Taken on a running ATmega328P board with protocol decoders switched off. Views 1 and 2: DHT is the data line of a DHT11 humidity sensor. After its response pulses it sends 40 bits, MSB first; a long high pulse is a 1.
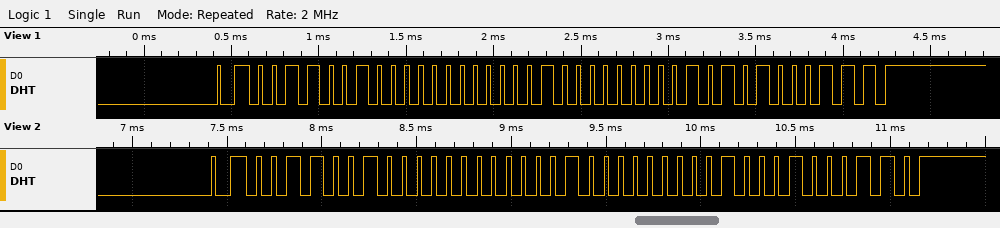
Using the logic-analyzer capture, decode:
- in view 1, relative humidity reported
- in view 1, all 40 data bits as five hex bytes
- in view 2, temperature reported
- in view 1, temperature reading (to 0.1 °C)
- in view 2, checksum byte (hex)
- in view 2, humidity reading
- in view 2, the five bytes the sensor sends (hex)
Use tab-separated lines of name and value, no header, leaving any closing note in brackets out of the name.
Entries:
in view 1, relative humidity reported	50 %
in view 1, all 40 data bits as five hex bytes	32 00 10 05 47
in view 2, temperature reported	16.4 °C
in view 1, temperature reading	16.5 °C
in view 2, checksum byte	0x46
in view 2, humidity reading	50 %
in view 2, the five bytes the sensor sends	32 00 10 04 46
